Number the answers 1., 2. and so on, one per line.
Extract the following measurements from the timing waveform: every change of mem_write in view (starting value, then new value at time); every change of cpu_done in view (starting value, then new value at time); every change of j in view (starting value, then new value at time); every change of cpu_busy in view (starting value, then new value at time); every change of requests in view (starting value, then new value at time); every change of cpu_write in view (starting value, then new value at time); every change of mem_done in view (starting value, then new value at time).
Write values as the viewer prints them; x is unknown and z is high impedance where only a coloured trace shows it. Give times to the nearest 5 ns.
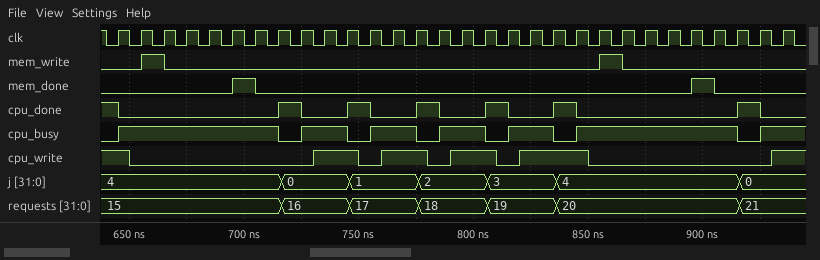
1. 0, 1 at 655 ns, 0 at 665 ns, 1 at 855 ns, 0 at 865 ns
2. 1, 0 at 645 ns, 1 at 715 ns, 0 at 725 ns, 1 at 745 ns, 0 at 755 ns, 1 at 775 ns, 0 at 785 ns, 1 at 805 ns, 0 at 815 ns, 1 at 835 ns, 0 at 845 ns, 1 at 915 ns, 0 at 925 ns
3. 4, 0 at 715 ns, 1 at 745 ns, 2 at 775 ns, 3 at 805 ns, 4 at 835 ns, 0 at 915 ns
4. 0, 1 at 645 ns, 0 at 715 ns, 1 at 725 ns, 0 at 745 ns, 1 at 755 ns, 0 at 775 ns, 1 at 785 ns, 0 at 805 ns, 1 at 815 ns, 0 at 835 ns, 1 at 845 ns, 0 at 915 ns, 1 at 925 ns
5. 15, 16 at 715 ns, 17 at 745 ns, 18 at 775 ns, 19 at 805 ns, 20 at 835 ns, 21 at 915 ns
6. 1, 0 at 650 ns, 1 at 730 ns, 0 at 750 ns, 1 at 760 ns, 0 at 780 ns, 1 at 790 ns, 0 at 810 ns, 1 at 820 ns, 0 at 850 ns, 1 at 930 ns
7. 0, 1 at 695 ns, 0 at 705 ns, 1 at 895 ns, 0 at 905 ns
